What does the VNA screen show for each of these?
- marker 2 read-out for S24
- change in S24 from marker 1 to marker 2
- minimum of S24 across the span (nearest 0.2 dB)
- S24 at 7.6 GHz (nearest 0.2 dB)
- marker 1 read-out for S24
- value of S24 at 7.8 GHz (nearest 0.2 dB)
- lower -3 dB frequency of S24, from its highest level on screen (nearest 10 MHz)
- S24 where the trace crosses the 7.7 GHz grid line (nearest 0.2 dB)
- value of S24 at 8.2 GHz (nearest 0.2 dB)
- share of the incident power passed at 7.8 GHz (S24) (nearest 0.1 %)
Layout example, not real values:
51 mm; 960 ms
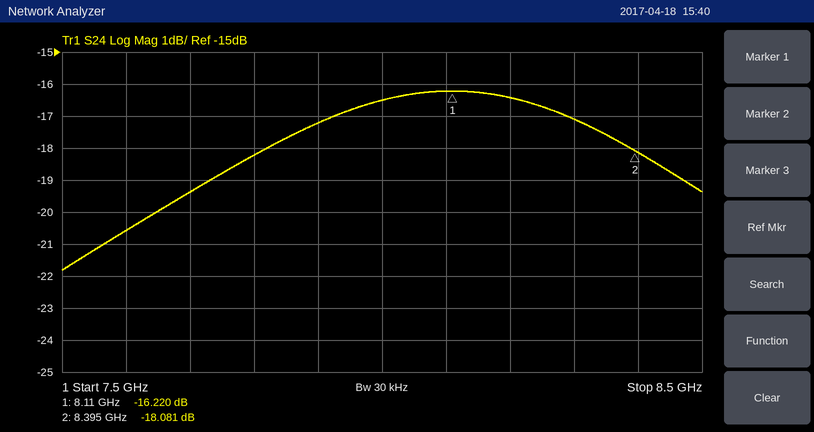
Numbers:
-18.081 dB; -1.861 dB; -21.8 dB; -20.6 dB; -16.220 dB; -18.2 dB; 7.71 GHz; -19.4 dB; -16.4 dB; 1.5 %
